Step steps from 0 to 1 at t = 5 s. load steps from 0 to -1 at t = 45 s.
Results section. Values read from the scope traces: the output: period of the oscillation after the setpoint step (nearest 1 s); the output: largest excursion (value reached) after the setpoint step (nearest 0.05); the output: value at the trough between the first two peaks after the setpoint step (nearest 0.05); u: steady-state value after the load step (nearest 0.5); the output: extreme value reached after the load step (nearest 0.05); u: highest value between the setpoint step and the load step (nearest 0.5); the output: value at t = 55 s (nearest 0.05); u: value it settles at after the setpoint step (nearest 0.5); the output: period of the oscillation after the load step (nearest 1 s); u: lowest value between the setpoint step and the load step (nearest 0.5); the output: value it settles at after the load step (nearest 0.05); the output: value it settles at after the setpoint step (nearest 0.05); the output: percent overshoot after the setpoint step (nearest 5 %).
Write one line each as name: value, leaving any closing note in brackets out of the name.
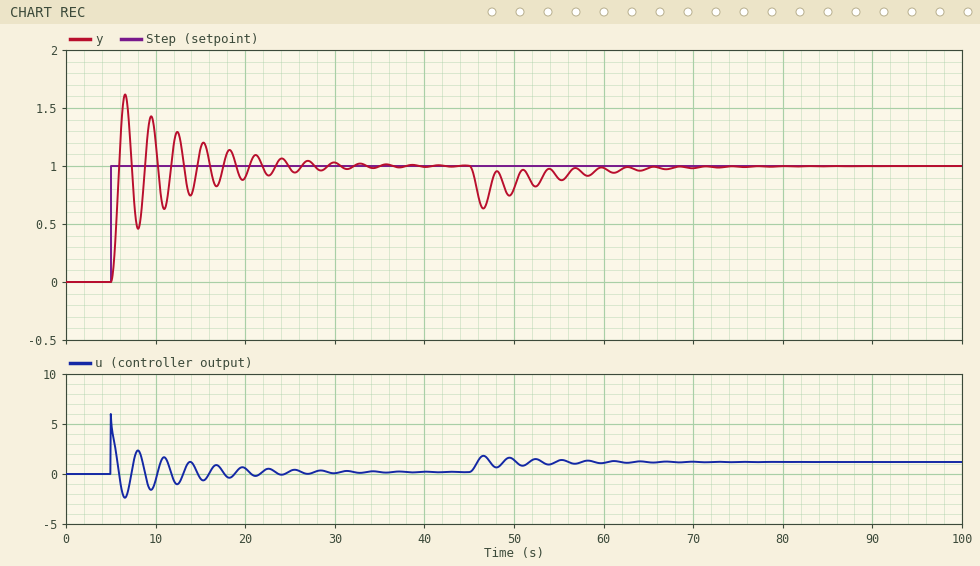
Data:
the output: period of the oscillation after the setpoint step: 3 s
the output: largest excursion (value reached) after the setpoint step: 1.60
the output: value at the trough between the first two peaks after the setpoint step: 0.45
u: steady-state value after the load step: 1.0
the output: extreme value reached after the load step: 0.65
u: highest value between the setpoint step and the load step: 6.0
the output: value at t = 55 s: 0.90
u: value it settles at after the setpoint step: 0.0
the output: period of the oscillation after the load step: 3 s
u: lowest value between the setpoint step and the load step: -2.5
the output: value it settles at after the load step: 1.00
the output: value it settles at after the setpoint step: 1.00
the output: percent overshoot after the setpoint step: 60 %
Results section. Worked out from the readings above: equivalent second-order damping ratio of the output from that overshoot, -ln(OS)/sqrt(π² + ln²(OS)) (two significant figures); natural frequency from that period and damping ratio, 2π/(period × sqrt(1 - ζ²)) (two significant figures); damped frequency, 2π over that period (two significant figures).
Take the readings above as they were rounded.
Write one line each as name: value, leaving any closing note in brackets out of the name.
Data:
equivalent second-order damping ratio of the output from that overshoot, -ln(OS)/sqrt(π² + ln²(OS)): 0.16
natural frequency from that period and damping ratio, 2π/(period × sqrt(1 - ζ²)): 2.1 rad/s
damped frequency, 2π over that period: 2.1 rad/s
